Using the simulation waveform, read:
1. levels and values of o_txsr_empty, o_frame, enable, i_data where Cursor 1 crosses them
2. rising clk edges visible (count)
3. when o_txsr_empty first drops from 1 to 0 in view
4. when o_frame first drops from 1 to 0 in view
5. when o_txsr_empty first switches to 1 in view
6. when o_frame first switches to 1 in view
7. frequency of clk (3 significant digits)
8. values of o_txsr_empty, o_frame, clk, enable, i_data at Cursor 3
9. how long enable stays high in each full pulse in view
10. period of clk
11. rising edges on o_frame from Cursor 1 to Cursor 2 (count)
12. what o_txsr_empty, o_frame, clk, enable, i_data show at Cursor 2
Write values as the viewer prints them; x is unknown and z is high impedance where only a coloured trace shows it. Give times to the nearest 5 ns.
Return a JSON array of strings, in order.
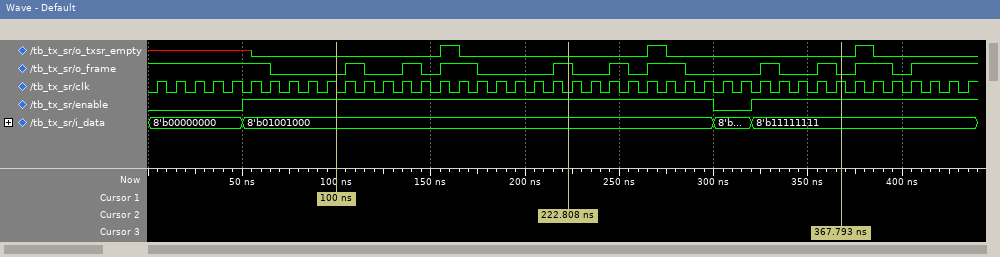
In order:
["o_txsr_empty=0, o_frame=0, enable=1, i_data=8'b01001000", "44", "165 ns", "65 ns", "155 ns", "105 ns", "100 MHz", "o_txsr_empty=0, o_frame=0, clk=1, enable=1, i_data=8'b11111111", "250 ns", "10 ns", "4", "o_txsr_empty=0, o_frame=1, clk=0, enable=1, i_data=8'b01001000"]
